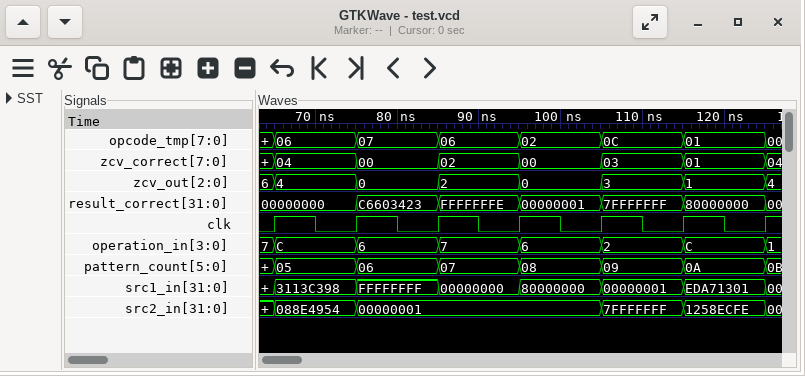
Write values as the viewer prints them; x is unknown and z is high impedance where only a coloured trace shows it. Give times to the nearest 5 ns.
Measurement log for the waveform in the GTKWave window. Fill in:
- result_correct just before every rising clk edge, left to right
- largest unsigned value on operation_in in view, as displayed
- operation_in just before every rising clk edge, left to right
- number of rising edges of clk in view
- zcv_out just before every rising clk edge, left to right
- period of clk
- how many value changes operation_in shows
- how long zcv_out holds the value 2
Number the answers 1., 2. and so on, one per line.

1. 00000000, 00000000, C6603423, FFFFFFFE, 00000001, 7FFFFFFF, 80000000
2. C
3. 7, C, 6, 7, 6, 2, C
4. 7
5. 6, 4, 0, 2, 0, 3, 1
6. 10 ns
7. 7
8. 10 ns
